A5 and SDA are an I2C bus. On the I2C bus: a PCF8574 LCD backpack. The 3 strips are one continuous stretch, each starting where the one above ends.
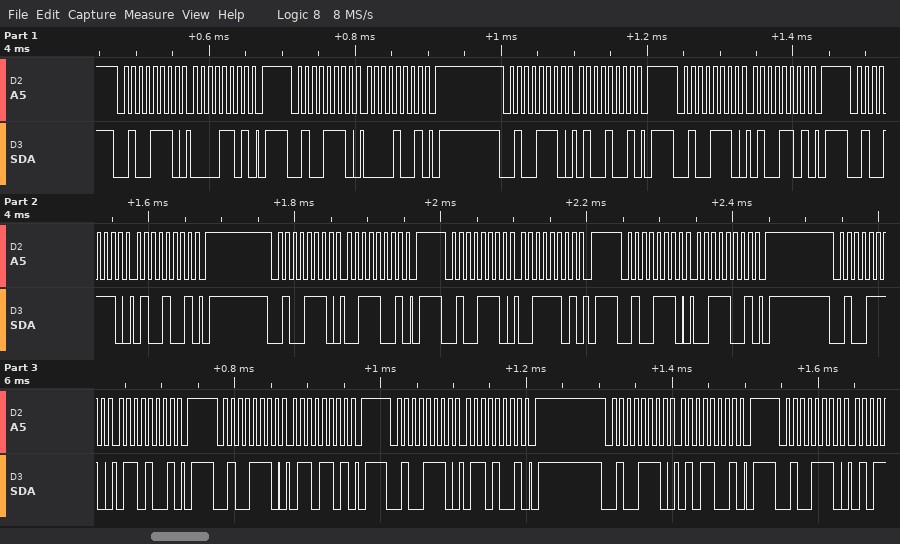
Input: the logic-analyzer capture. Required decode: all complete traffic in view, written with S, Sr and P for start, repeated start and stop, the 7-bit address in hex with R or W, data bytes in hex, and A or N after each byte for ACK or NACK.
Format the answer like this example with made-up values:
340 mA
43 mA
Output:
S 27W A 0D A P S 27W A 09 A P S 27W A 49 A P S 27W A 4D A P S 27W A 49 A P S 27W A 39 A P S 27W A 3D A P S 27W A 39 A P S 27W A 69 A P S 27W A 6D A P S 27W A 69 A P S 27W A 59 A P S 27W A
